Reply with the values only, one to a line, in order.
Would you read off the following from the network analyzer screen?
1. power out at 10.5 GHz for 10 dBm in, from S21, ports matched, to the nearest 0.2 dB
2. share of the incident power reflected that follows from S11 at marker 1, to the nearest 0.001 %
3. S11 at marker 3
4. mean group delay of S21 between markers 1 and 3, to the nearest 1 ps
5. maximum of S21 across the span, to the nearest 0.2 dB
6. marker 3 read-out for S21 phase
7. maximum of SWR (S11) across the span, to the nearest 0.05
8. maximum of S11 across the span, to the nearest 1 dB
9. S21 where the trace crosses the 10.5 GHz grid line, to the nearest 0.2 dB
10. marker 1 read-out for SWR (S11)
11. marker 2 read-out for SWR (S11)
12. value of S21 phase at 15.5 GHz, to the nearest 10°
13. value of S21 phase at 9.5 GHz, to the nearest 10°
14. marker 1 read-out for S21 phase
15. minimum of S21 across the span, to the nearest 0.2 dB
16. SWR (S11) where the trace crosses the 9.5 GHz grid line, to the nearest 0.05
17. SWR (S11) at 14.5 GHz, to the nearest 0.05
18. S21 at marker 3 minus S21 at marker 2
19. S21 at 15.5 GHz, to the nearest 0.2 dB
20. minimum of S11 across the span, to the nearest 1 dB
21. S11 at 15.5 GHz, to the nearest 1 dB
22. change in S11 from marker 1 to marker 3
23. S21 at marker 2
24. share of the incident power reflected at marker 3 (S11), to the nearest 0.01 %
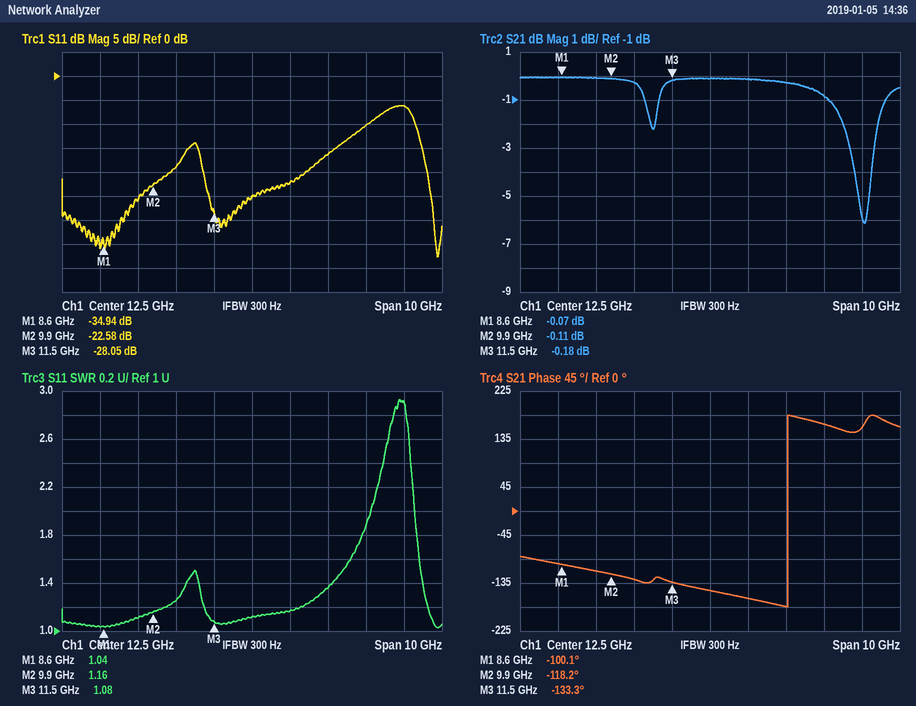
9.8 dBm
0.032 %
-28.05 dB
32 ps
0.0 dB
-133.3°
2.95
-6 dB
-0.2 dB
1.04
1.16
160°
-110°
-100.1°
-6.2 dB
1.10
1.35
-0.07 dB
-0.8 dB
-38 dB
-10 dB
6.89 dB
-0.11 dB
0.16 %
